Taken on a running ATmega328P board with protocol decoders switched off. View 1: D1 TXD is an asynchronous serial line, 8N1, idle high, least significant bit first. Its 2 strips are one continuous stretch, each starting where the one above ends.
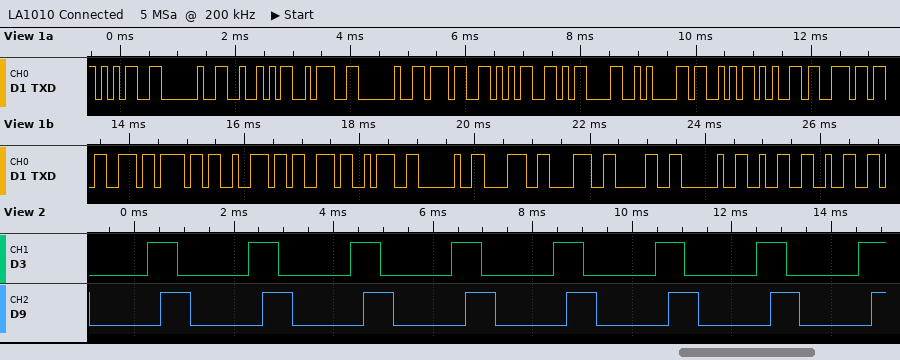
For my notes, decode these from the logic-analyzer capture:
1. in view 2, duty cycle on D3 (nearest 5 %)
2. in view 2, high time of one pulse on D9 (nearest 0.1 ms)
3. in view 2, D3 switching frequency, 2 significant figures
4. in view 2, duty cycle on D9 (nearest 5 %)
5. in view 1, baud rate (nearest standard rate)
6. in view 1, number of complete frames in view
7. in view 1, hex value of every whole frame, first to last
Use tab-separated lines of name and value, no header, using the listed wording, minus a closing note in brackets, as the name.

in view 2, duty cycle on D3	30 %
in view 2, high time of one pulse on D9	0.6 ms
in view 2, D3 switching frequency, 2 significant figures	490 Hz
in view 2, duty cycle on D9	30 %
in view 1, baud rate	9600 baud
in view 1, number of complete frames in view	24
in view 1, hex value of every whole frame, first to last	35 20 52 3A 20 37 35 0D 0A 53 65 6E 73 6F 72 73 3A 20 38 38 30 20 32 32
